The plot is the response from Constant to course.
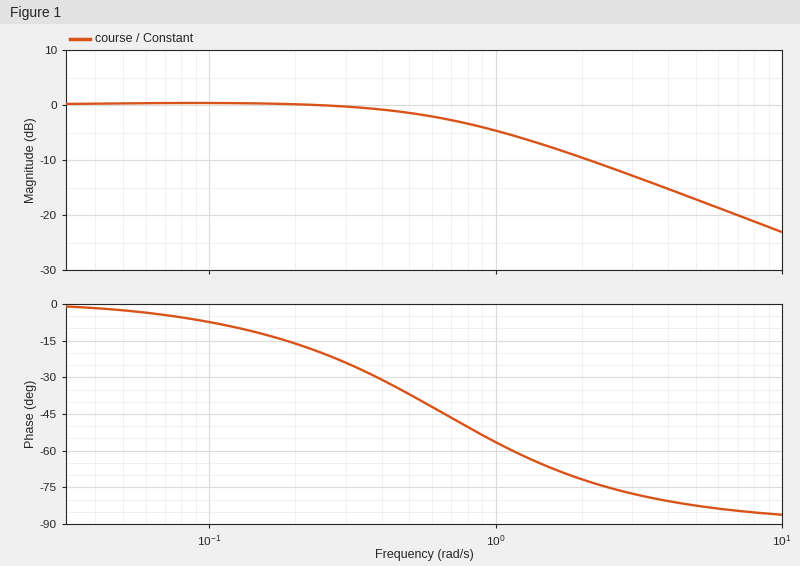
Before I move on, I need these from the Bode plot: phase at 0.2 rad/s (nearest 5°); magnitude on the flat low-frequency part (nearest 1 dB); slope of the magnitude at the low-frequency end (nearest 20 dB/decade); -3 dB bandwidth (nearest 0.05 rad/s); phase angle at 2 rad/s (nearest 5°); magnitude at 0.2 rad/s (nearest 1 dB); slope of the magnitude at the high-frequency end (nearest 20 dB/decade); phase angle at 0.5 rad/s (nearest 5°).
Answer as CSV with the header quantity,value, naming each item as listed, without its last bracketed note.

quantity,value
phase at 0.2 rad/s,-15°
magnitude on the flat low-frequency part,0 dB
slope of the magnitude at the low-frequency end,0 dB/decade
-3 dB bandwidth,0.70 rad/s
phase angle at 2 rad/s,-70°
magnitude at 0.2 rad/s,0 dB
slope of the magnitude at the high-frequency end,-20 dB/decade
phase angle at 0.5 rad/s,-35°
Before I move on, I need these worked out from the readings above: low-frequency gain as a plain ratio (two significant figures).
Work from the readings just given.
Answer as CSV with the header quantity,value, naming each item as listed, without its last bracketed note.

quantity,value
low-frequency gain as a plain ratio,1.0
